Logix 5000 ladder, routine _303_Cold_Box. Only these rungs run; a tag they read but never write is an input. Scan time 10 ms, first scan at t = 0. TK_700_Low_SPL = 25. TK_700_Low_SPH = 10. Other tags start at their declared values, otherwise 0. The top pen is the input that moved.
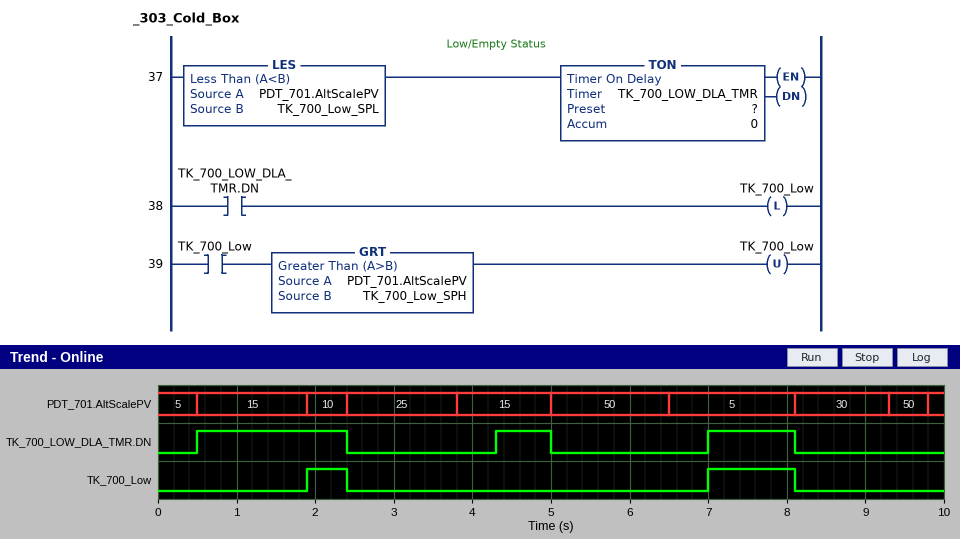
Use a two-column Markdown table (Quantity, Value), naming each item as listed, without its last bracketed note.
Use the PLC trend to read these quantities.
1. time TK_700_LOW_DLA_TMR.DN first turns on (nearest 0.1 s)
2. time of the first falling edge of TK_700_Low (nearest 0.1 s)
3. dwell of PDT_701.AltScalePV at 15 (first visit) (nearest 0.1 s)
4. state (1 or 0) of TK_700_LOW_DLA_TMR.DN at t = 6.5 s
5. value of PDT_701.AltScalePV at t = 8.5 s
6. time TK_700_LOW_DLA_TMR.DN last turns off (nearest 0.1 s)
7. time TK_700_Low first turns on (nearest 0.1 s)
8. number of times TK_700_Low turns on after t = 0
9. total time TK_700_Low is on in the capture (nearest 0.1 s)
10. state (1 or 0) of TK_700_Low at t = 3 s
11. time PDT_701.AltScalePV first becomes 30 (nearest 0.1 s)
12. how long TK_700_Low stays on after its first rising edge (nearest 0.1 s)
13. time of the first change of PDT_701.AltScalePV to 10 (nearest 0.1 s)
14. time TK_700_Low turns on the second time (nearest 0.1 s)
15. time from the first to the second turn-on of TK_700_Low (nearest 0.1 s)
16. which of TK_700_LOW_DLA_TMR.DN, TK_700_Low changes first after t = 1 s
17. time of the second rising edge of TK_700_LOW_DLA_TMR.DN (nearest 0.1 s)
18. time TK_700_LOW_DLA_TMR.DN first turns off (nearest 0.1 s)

| Quantity | Value |
|---|---|
| time TK_700_LOW_DLA_TMR.DN first turns on | 0.5 s |
| time of the first falling edge of TK_700_Low | 2.4 s |
| dwell of PDT_701.AltScalePV at 15 (first visit) | 1.4 s |
| state (1 or 0) of TK_700_LOW_DLA_TMR.DN at t = 6.5 s | 0 |
| value of PDT_701.AltScalePV at t = 8.5 s | 30 |
| time TK_700_LOW_DLA_TMR.DN last turns off | 8.1 s |
| time TK_700_Low first turns on | 1.9 s |
| number of times TK_700_Low turns on after t = 0 | 2 |
| total time TK_700_Low is on in the capture | 1.6 s |
| state (1 or 0) of TK_700_Low at t = 3 s | 0 |
| time PDT_701.AltScalePV first becomes 30 | 8.1 s |
| how long TK_700_Low stays on after its first rising edge | 0.5 s |
| time of the first change of PDT_701.AltScalePV to 10 | 1.9 s |
| time TK_700_Low turns on the second time | 7.0 s |
| time from the first to the second turn-on of TK_700_Low | 5.1 s |
| which of TK_700_LOW_DLA_TMR.DN, TK_700_Low changes first after t = 1 s | TK_700_Low |
| time of the second rising edge of TK_700_LOW_DLA_TMR.DN | 4.3 s |
| time TK_700_LOW_DLA_TMR.DN first turns off | 2.4 s |
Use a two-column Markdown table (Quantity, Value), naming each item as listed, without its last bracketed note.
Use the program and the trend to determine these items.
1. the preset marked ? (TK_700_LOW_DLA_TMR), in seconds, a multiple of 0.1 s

| Quantity | Value |
|---|---|
| the preset marked ? (TK_700_LOW_DLA_TMR), in seconds, a multiple of 0.1 s | 0.5 s |
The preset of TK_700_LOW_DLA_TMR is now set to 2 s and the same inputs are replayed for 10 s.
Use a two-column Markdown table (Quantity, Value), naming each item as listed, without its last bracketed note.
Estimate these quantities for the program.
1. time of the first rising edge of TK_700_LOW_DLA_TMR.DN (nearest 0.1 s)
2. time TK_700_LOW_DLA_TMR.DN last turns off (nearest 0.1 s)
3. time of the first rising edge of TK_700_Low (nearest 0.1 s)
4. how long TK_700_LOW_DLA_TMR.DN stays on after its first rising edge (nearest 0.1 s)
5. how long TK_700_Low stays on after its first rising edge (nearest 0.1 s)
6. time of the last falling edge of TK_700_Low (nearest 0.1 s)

| Quantity | Value |
|---|---|
| time of the first rising edge of TK_700_LOW_DLA_TMR.DN | 2.0 s |
| time TK_700_LOW_DLA_TMR.DN last turns off | 2.4 s |
| time of the first rising edge of TK_700_Low | 2.0 s |
| how long TK_700_LOW_DLA_TMR.DN stays on after its first rising edge | 0.4 s |
| how long TK_700_Low stays on after its first rising edge | 0.4 s |
| time of the last falling edge of TK_700_Low | 2.4 s |
